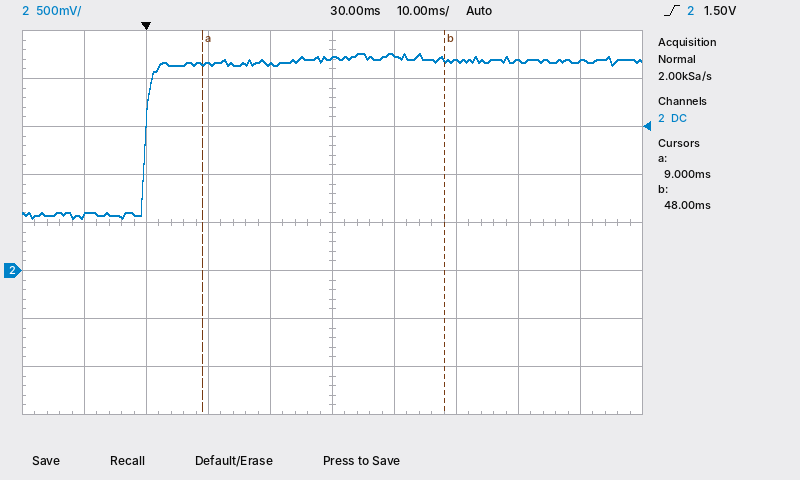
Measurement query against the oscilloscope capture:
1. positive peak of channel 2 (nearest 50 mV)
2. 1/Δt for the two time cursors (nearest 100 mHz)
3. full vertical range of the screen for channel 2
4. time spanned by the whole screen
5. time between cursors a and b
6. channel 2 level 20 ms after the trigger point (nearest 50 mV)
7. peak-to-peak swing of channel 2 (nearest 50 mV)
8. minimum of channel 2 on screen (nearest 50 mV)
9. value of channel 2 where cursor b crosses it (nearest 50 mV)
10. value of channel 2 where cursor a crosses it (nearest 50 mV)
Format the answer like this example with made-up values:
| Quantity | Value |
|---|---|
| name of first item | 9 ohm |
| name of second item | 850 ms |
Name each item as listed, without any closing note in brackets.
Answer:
| Quantity | Value |
|---|---|
| positive peak of channel 2 | 2.25 V |
| 1/Δt for the two time cursors | 25.6 Hz |
| full vertical range of the screen for channel 2 | 4 V |
| time spanned by the whole screen | 100 ms |
| time between cursors a and b | 39 ms |
| channel 2 level 20 ms after the trigger point | 2.15 V |
| peak-to-peak swing of channel 2 | 1.70 V |
| minimum of channel 2 on screen | 550 mV |
| value of channel 2 where cursor b crosses it | 2.20 V |
| value of channel 2 where cursor a crosses it | 2.15 V |
